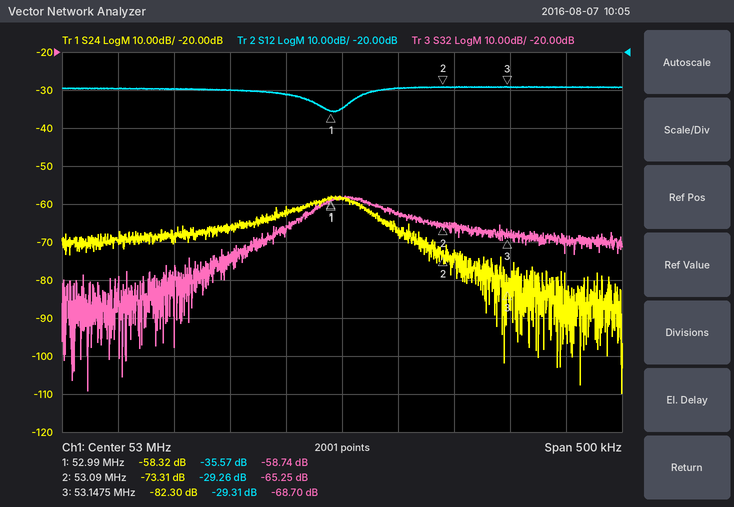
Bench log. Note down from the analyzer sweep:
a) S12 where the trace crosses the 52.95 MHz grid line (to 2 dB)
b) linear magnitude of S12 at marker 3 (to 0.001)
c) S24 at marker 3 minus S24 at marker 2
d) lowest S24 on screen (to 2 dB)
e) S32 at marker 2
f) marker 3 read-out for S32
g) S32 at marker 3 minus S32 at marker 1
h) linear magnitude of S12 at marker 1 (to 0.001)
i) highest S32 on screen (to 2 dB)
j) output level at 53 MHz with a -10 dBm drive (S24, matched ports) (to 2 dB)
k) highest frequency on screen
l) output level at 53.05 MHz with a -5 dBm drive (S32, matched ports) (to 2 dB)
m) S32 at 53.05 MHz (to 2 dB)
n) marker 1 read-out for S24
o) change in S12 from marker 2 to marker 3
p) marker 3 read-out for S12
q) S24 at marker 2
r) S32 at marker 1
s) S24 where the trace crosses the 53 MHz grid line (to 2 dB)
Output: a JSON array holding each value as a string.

["-32 dB", "0.034", "-8.99 dB", "-110 dB", "-65.25 dB", "-68.70 dB", "-9.96 dB", "0.017", "-58 dB", "-68 dBm", "53.25 MHz", "-68 dBm", "-62 dB", "-58.32 dB", "-0.05 dB", "-29.31 dB", "-73.31 dB", "-58.74 dB", "-58 dB"]
